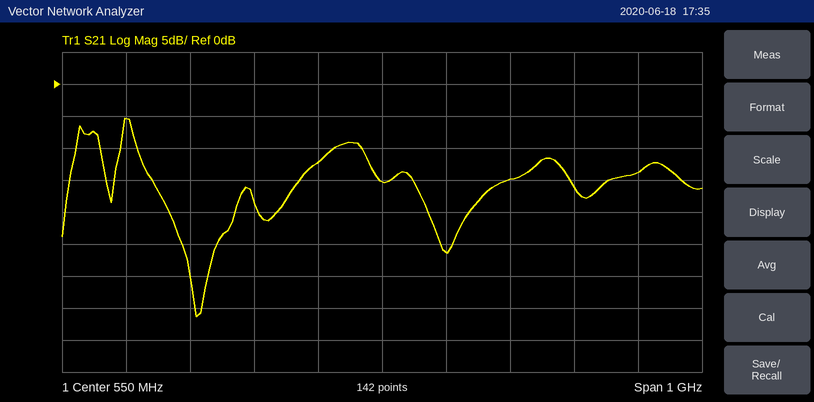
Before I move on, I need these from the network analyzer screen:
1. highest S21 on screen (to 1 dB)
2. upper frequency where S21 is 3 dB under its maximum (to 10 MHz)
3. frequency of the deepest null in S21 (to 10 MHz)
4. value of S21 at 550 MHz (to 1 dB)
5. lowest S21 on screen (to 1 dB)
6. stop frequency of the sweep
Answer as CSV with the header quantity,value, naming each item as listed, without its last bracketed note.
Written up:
quantity,value
highest S21 on screen,-5 dB
upper frequency where S21 is 3 dB under its maximum,160 MHz
frequency of the deepest null in S21,260 MHz
value of S21 at 550 MHz,-15 dB
lowest S21 on screen,-36 dB
stop frequency of the sweep,1.05 GHz
